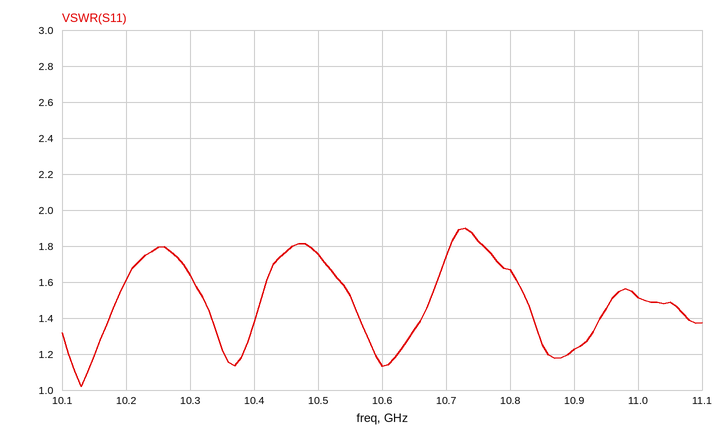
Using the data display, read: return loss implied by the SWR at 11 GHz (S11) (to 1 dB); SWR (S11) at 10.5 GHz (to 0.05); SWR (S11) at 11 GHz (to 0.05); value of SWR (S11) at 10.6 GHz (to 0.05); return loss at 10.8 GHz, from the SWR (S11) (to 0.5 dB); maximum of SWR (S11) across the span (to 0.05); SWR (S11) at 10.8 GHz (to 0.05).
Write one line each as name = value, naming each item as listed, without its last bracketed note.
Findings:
return loss implied by the SWR at 11 GHz (S11) = 14 dB
SWR (S11) at 10.5 GHz = 1.75
SWR (S11) at 11 GHz = 1.50
value of SWR (S11) at 10.6 GHz = 1.15
return loss at 10.8 GHz, from the SWR (S11) = 12.0 dB
maximum of SWR (S11) across the span = 1.90
SWR (S11) at 10.8 GHz = 1.65
